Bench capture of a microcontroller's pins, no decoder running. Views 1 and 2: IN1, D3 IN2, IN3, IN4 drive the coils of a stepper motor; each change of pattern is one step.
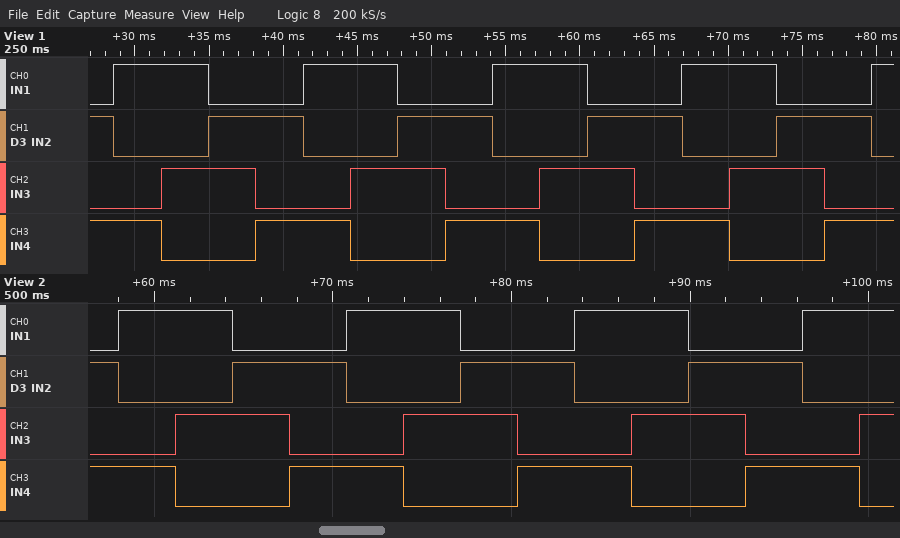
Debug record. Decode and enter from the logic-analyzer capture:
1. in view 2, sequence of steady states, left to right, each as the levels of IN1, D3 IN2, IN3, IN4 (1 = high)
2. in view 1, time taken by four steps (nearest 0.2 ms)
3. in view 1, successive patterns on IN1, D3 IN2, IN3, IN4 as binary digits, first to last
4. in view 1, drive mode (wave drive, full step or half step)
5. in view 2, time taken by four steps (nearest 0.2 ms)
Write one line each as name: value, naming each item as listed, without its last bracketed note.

in view 2, sequence of steady states, left to right, each as the levels of IN1, D3 IN2, IN3, IN4: 0101 1001 1010 0110 0101 1001 1010 0110 0101 1001 1010 0110 0101 1001 1010
in view 1, time taken by four steps: 12.8 ms
in view 1, successive patterns on IN1, D3 IN2, IN3, IN4 as binary digits, first to last: 0101 1001 1010 0110 0101 1001 1010 0110 0101 1001 1010 0110 0101 1001 1010 0110 0101 1001
in view 1, drive mode: full step
in view 2, time taken by four steps: 12.8 ms
